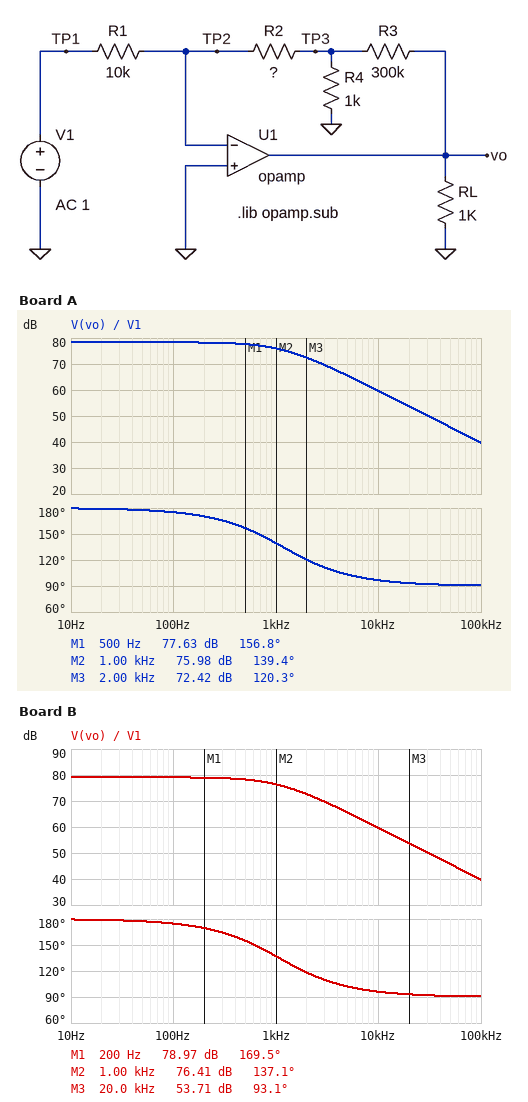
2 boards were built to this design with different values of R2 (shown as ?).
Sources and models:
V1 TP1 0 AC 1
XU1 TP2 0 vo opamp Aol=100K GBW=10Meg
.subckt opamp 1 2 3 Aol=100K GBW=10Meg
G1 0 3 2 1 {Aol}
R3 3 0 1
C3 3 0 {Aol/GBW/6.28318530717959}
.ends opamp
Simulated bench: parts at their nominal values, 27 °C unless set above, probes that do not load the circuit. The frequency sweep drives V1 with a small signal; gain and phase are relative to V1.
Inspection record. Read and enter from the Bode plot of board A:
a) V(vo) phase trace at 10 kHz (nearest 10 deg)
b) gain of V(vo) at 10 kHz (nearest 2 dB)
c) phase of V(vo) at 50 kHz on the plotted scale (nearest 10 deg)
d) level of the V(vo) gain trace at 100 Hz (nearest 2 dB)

100 deg
60 dB
90 deg
78 dB
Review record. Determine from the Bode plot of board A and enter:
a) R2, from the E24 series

300 kΩ
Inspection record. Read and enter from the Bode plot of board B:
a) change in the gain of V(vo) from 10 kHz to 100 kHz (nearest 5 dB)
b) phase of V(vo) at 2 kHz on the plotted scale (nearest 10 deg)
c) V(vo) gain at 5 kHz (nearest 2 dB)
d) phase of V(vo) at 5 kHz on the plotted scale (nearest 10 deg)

-20 dB
120 deg
66 dB
100 deg
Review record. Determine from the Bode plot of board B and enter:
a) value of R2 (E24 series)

330 kΩ
